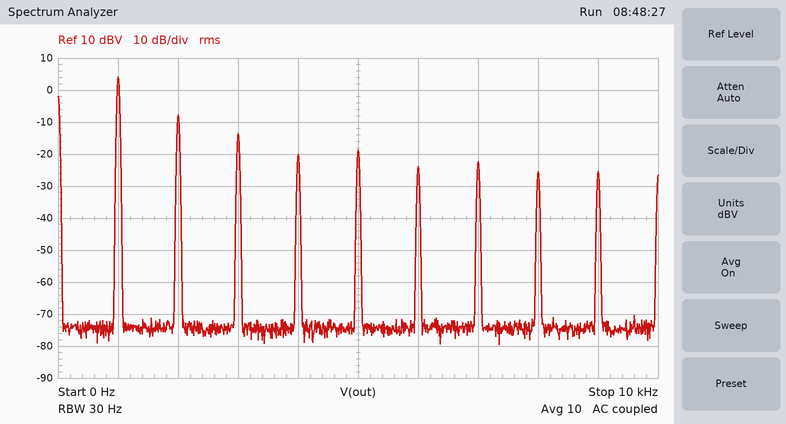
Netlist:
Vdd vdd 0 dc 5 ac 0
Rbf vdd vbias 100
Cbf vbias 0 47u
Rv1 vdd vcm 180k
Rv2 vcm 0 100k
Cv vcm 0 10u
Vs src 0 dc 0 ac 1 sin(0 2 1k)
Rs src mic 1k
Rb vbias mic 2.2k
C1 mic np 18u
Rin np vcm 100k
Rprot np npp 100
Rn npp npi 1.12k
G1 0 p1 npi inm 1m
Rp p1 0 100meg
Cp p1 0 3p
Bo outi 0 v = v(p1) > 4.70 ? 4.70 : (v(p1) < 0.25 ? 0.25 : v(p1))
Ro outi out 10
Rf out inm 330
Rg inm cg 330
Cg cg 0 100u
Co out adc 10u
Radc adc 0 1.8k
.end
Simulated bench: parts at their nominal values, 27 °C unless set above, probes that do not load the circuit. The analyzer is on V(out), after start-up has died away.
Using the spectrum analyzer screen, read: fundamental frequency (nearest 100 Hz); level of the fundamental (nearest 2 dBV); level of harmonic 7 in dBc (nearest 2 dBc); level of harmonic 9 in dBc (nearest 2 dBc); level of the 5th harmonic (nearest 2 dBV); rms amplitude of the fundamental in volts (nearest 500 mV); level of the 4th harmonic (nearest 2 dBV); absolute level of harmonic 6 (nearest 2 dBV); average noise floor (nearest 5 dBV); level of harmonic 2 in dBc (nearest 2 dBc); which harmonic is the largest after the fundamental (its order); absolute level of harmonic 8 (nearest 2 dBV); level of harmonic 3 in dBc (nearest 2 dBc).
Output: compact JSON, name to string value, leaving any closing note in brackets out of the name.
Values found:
{"fundamental frequency": "1.0 kHz", "level of the fundamental": "4 dBV", "level of harmonic 7 in dBc": "-26 dBc", "level of harmonic 9 in dBc": "-30 dBc", "level of the 5th harmonic": "-18 dBV", "rms amplitude of the fundamental in volts": "1.5 V", "level of the 4th harmonic": "-20 dBV", "absolute level of harmonic 6": "-24 dBV", "average noise floor": "-75 dBV", "level of harmonic 2 in dBc": "-12 dBc", "which harmonic is the largest after the fundamental": "2", "absolute level of harmonic 8": "-26 dBV", "level of harmonic 3 in dBc": "-18 dBc"}
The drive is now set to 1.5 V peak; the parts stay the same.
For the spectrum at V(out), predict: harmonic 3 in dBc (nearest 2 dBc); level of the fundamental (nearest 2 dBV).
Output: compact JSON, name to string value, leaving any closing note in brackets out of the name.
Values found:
{"harmonic 3 in dBc": "-20 dBc", "level of the fundamental": "2 dBV"}
